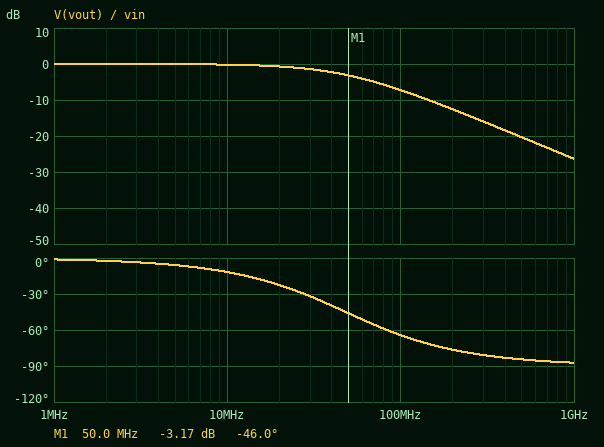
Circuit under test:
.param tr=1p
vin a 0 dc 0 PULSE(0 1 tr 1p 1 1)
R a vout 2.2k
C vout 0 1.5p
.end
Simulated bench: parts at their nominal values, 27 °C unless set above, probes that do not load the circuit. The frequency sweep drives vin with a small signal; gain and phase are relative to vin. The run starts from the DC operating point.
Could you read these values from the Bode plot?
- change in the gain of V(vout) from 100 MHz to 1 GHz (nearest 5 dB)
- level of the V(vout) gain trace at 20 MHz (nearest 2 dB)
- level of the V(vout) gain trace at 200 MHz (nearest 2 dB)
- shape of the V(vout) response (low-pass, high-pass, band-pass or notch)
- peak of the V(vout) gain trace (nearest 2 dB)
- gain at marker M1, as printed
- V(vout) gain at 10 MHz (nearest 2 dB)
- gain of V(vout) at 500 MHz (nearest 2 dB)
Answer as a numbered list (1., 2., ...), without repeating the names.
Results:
1. -20 dB
2. 0 dB
3. -12 dB
4. low-pass
5. 0 dB
6. -3.17 dB
7. 0 dB
8. -20 dB
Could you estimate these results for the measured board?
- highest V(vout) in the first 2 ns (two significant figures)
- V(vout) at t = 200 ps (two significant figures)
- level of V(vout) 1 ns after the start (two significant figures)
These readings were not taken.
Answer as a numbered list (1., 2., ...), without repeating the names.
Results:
1. 450 mV
2. 58 mV
3. 260 mV
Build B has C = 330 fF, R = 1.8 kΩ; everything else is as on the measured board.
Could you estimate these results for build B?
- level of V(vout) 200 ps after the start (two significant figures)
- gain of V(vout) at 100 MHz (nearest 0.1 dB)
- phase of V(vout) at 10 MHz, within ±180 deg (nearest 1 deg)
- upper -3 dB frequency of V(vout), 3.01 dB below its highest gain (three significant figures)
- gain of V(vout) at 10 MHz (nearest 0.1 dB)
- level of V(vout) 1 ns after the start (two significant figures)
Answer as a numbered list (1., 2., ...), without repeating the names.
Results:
1. 280 mV
2. -0.6 dB
3. -2 deg
4. 268 MHz
5. 0 dB
6. 810 mV
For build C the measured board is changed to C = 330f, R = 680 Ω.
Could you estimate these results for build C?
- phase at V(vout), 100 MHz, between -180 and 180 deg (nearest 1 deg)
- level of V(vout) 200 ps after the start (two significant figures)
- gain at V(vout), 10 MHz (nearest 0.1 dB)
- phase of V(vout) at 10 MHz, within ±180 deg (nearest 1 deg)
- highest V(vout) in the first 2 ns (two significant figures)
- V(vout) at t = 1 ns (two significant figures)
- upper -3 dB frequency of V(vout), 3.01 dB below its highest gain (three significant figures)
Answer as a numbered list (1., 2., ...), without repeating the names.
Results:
1. -8 deg
2. 590 mV
3. 0 dB
4. -1 deg
5. 1.0 V
6. 990 mV
7. 709 MHz
